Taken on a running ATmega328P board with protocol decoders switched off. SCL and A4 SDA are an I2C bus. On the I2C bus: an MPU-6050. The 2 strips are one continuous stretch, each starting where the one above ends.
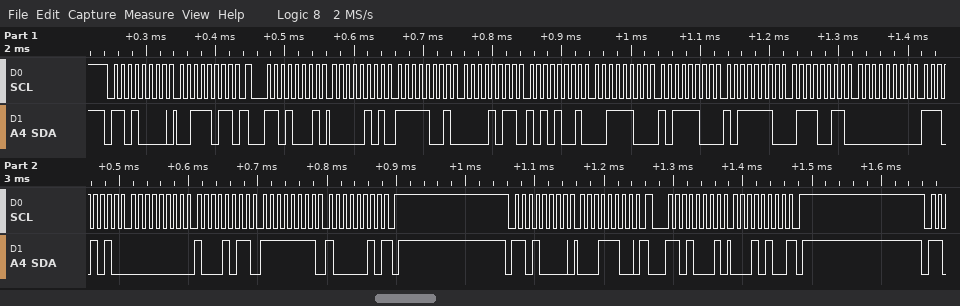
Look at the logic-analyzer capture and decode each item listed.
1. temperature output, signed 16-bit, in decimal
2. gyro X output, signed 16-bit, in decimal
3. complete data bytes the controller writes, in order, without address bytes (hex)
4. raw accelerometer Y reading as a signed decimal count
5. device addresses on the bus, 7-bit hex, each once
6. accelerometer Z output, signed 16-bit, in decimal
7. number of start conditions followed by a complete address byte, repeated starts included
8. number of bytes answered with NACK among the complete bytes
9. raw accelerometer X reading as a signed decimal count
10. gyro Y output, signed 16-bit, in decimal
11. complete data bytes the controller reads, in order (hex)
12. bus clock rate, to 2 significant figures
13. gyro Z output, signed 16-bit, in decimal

-16781
234
3B 1C
2985
0x68
15548
4
2
1529
139
05 F9 0B A9 3C BC BE 73 00 EA 00 8B FF 82 14
100 kHz
-126
